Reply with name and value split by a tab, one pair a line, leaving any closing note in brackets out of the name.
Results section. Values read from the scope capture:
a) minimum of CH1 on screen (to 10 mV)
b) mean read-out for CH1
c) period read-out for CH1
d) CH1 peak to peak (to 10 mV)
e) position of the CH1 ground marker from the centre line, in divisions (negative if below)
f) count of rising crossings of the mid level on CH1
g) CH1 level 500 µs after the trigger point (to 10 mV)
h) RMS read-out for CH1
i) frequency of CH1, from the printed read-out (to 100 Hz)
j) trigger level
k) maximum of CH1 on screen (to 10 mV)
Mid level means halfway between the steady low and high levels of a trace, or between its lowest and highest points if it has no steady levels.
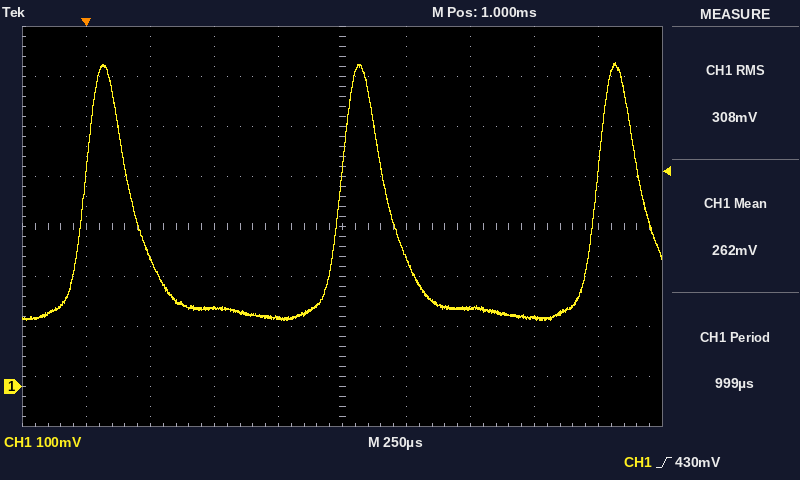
minimum of CH1 on screen	130 mV
mean read-out for CH1	262 mV
period read-out for CH1	999 µs
CH1 peak to peak	520 mV
position of the CH1 ground marker from the centre line, in divisions	-3.2 div
count of rising crossings of the mid level on CH1	3
CH1 level 500 µs after the trigger point	160 mV
RMS read-out for CH1	308 mV
frequency of CH1, from the printed read-out	1.0 kHz
trigger level	430 mV
maximum of CH1 on screen	650 mV
